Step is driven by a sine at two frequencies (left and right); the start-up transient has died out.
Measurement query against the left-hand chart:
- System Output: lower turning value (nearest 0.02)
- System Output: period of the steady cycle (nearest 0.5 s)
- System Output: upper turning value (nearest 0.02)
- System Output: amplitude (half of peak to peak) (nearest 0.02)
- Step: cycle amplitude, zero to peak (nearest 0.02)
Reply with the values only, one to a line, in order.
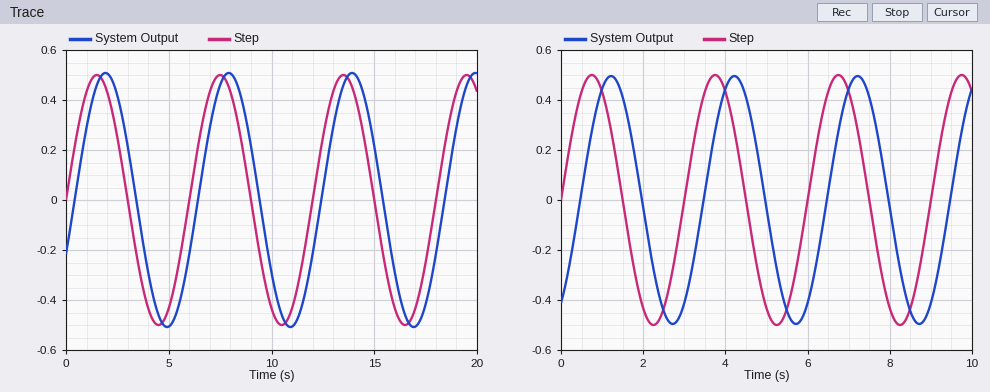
-0.50
6.0 s
0.50
0.50
0.50
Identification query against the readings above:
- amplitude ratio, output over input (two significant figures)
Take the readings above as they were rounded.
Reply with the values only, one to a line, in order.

1.0
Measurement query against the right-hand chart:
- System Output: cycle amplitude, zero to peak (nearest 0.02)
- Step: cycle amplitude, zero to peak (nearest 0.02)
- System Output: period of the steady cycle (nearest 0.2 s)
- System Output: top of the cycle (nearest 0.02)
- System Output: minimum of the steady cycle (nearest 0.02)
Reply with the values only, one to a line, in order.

0.50
0.50
3.0 s
0.50
-0.50
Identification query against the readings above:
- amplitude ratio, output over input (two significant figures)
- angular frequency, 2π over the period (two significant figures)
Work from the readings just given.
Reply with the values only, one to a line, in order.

1.0
2.1 rad/s
